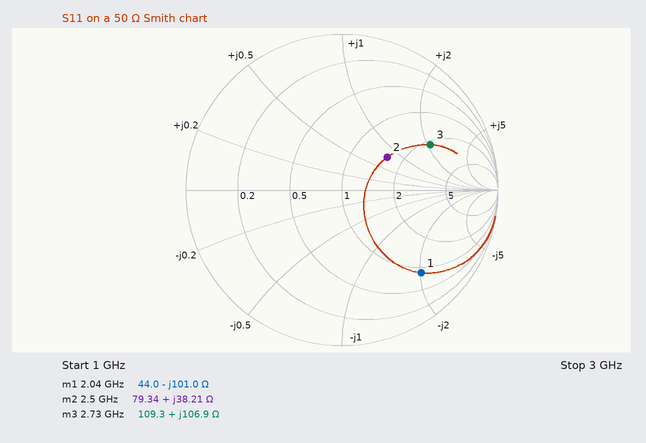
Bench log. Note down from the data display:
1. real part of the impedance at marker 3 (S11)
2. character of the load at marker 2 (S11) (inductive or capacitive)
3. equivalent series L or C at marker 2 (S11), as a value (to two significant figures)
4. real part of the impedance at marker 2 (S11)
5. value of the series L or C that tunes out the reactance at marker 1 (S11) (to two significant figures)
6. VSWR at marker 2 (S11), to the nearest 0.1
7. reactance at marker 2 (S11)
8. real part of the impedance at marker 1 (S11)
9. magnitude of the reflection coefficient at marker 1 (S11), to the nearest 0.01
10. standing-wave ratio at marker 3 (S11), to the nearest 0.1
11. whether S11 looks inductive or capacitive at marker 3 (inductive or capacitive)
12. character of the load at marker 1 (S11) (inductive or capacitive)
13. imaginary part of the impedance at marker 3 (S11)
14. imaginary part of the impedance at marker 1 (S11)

109.3 Ω
inductive
2.4 nH
79.34 Ω
7.9 nH
2.1
+38.21 Ω
44.0 Ω
0.73
4.5
inductive
capacitive
+106.9 Ω
-101.0 Ω
